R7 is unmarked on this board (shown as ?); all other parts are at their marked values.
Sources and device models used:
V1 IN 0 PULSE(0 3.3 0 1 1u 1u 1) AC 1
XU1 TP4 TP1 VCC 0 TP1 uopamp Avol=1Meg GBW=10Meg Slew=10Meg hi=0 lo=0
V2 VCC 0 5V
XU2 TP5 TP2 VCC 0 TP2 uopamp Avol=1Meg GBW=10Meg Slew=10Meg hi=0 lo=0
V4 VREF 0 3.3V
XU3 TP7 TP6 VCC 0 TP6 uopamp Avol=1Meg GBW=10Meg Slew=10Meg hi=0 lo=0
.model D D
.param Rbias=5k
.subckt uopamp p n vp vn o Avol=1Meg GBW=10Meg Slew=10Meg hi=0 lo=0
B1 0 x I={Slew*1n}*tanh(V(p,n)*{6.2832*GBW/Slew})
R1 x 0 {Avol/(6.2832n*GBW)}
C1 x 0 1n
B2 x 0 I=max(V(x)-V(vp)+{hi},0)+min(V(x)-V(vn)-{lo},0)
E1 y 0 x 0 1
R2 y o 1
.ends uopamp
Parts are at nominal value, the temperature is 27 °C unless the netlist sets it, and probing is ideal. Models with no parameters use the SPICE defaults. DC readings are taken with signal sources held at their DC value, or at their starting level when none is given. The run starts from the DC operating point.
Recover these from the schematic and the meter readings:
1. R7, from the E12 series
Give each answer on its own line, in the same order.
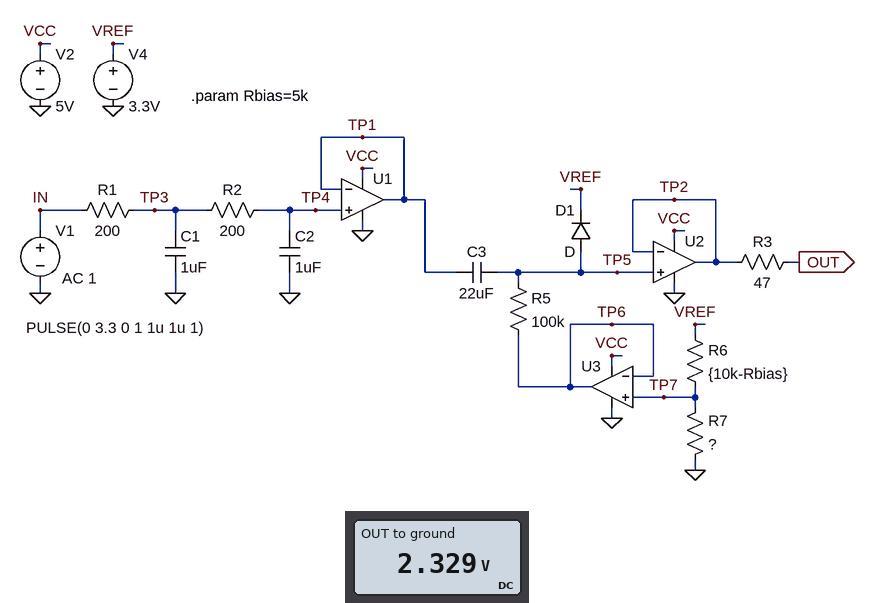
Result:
12 kΩ
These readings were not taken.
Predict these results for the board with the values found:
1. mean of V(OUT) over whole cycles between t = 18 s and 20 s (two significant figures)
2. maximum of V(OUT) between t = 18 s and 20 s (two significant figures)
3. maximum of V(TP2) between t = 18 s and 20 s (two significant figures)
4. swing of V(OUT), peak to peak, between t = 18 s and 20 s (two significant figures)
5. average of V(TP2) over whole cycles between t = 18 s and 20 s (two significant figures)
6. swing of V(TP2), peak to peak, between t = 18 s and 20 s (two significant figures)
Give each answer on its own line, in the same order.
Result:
2.3 V
3.8 V
3.8 V
3.3 V
2.3 V
3.3 V
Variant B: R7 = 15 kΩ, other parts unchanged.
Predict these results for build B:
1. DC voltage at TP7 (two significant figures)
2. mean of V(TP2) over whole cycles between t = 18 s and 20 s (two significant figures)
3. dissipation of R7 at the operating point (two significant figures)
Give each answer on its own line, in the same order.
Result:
2.5 V
2.4 V
410 µW
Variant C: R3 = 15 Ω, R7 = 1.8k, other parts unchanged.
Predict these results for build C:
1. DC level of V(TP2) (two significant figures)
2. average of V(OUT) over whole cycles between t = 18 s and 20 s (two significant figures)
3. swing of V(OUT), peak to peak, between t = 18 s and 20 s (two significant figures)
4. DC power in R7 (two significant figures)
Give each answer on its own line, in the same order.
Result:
870 mV
970 mV
2.4 V
420 µW
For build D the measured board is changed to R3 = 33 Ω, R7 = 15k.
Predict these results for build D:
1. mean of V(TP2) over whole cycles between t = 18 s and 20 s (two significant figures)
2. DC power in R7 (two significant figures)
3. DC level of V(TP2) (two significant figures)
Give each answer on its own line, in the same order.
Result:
2.4 V
410 µW
2.5 V
